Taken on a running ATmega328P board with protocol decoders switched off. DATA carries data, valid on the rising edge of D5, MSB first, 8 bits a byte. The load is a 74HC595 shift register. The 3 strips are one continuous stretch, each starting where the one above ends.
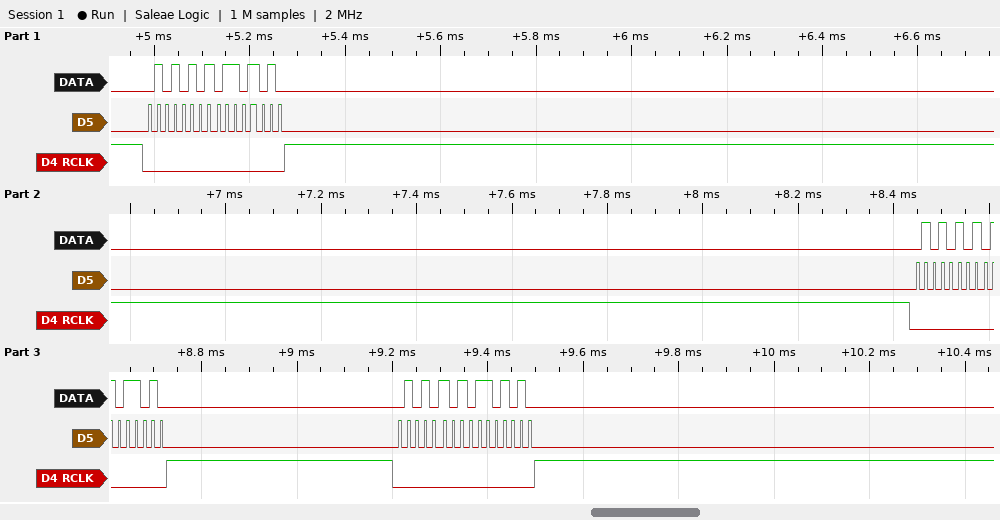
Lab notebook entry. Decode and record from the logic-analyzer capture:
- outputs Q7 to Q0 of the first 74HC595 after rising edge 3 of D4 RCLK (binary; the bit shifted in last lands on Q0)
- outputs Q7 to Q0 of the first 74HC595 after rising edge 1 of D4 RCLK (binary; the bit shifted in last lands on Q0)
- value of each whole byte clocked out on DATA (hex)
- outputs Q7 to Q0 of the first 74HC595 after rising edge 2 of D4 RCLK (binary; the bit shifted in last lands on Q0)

01101010
01101010
0x55 0x6A 0x55 0x5A 0x55 0x6A
01011010
